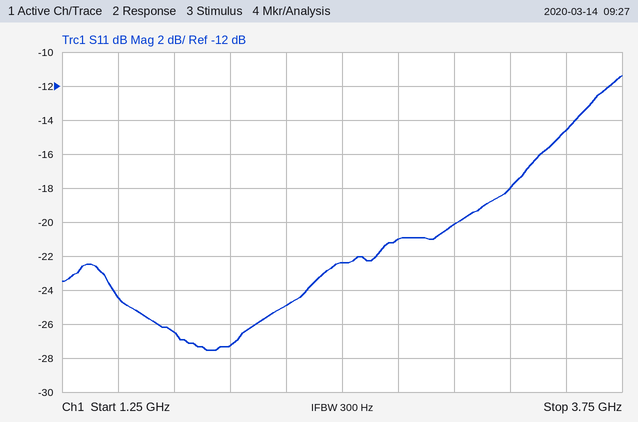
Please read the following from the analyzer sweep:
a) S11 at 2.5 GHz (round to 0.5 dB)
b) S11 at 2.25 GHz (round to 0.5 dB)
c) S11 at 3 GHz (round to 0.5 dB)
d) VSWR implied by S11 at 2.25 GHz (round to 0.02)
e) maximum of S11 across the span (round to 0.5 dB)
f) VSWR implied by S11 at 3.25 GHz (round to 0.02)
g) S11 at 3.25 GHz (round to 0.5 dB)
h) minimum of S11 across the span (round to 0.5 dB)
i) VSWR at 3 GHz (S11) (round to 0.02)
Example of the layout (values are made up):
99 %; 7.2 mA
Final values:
-22.5 dB; -25.0 dB; -20.0 dB; 1.12; -11.5 dB; 1.28; -18.0 dB; -27.5 dB; 1.22
